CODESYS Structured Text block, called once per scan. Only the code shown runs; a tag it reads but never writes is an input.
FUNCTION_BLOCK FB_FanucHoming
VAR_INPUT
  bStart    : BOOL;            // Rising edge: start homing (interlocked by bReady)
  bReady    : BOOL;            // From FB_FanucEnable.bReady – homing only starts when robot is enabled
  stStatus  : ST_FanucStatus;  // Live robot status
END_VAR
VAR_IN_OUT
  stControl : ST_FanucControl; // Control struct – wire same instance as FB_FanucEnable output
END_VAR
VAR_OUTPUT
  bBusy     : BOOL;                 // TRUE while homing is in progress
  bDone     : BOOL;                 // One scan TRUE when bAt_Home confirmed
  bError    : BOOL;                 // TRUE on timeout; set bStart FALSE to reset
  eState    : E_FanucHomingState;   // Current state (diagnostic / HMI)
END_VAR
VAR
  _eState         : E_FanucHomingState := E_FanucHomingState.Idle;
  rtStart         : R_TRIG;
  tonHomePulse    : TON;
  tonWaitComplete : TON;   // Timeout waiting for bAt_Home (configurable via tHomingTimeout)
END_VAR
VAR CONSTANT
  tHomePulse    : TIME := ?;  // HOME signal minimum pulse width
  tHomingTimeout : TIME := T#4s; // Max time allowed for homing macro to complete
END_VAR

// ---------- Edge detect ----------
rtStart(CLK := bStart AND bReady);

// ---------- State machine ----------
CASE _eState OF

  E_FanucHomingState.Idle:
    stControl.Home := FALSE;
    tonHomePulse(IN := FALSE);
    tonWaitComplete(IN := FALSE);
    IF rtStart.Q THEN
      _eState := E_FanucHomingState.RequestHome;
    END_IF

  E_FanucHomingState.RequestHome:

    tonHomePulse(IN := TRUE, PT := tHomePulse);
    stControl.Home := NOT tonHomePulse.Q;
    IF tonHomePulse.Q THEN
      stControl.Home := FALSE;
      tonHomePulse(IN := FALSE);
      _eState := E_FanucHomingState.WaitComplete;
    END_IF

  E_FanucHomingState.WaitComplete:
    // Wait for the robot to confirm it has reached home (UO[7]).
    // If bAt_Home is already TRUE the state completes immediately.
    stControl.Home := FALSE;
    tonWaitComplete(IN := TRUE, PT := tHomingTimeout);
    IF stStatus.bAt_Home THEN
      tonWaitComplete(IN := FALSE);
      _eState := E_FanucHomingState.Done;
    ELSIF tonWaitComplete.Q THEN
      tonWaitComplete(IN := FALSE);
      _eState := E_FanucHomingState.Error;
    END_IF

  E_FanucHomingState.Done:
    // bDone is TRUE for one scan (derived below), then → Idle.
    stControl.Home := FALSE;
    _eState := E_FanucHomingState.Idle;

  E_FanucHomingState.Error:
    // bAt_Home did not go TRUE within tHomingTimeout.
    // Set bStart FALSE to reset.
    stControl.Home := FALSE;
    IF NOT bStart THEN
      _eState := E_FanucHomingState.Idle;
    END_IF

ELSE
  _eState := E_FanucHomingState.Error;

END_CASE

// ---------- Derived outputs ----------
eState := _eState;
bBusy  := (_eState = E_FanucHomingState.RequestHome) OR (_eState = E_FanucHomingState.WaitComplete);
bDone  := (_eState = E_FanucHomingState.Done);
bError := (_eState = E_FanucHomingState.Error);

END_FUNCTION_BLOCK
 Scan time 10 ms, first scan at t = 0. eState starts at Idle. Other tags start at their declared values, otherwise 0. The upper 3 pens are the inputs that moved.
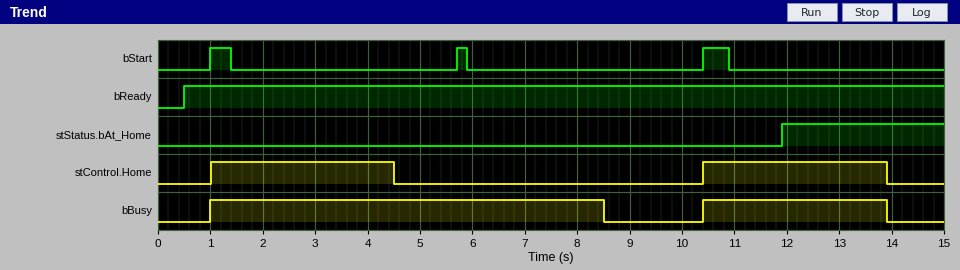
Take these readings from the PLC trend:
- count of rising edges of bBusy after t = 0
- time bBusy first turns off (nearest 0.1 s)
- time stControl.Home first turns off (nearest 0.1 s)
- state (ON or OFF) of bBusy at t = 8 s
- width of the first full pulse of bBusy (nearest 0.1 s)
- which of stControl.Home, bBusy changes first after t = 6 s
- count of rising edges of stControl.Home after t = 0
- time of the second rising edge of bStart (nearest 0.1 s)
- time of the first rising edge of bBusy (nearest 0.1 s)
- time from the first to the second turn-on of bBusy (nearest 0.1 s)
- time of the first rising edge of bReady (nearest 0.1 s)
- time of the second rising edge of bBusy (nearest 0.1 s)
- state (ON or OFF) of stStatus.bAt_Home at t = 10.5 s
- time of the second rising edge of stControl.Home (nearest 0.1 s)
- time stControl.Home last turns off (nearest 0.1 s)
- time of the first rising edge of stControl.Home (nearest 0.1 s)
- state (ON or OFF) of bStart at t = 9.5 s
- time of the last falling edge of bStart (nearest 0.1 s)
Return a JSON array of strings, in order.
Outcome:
["2", "8.5 s", "4.5 s", "ON", "7.5 s", "bBusy", "2", "5.7 s", "1.0 s", "9.4 s", "0.5 s", "10.4 s", "OFF", "10.4 s", "13.9 s", "1.0 s", "OFF", "10.9 s"]
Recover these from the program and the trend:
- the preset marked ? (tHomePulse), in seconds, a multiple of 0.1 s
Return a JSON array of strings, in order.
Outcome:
["3.5 s"]
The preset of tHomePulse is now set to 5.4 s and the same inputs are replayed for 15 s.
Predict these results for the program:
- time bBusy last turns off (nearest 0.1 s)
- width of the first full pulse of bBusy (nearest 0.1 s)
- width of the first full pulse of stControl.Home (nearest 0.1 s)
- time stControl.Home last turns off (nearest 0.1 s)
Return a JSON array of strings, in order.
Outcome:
["10.4 s", "9.4 s", "5.4 s", "6.4 s"]
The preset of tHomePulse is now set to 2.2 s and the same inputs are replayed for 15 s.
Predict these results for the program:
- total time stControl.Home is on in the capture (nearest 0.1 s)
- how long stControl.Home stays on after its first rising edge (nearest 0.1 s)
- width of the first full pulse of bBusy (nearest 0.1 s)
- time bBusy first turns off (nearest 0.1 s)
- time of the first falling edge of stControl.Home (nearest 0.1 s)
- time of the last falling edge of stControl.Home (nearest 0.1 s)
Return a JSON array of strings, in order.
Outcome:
["4.4 s", "2.2 s", "6.2 s", "7.2 s", "3.2 s", "12.6 s"]
